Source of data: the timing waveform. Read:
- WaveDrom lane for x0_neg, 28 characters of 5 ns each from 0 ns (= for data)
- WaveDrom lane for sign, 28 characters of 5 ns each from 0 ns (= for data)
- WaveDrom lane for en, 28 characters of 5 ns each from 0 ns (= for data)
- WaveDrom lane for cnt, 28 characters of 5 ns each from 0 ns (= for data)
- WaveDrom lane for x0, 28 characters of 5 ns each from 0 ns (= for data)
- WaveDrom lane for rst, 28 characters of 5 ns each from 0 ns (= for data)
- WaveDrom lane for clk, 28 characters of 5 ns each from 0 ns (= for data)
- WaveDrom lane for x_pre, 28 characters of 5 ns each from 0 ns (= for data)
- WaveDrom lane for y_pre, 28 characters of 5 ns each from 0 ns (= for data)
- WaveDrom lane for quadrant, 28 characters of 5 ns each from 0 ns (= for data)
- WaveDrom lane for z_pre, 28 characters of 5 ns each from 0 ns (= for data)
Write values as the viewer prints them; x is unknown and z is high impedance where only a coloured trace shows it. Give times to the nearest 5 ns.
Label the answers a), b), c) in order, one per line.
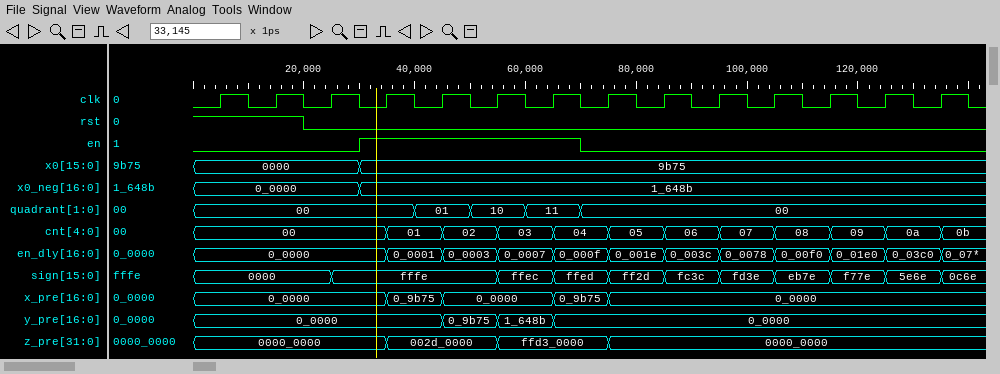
a) {name: 'x0_neg', wave: '=.....=.....................', data: '0_0000 1_648b'}
b) {name: 'sign', wave: '=....=.....=.=.=.=.=.=.=.=.=', data: '0000 fffe ffec ffed ff2d fc3c fd3e eb7e f77e 5e6e 0c6e'}
c) {name: 'en', wave: '0.....1.......0.............'}
d) {name: 'cnt', wave: '=......=.=.=.=.=.=.=.=.=.=.=', data: '00 01 02 03 04 05 06 07 08 09 0a 0b'}
e) {name: 'x0', wave: '=.....=.....................', data: '0000 9b75'}
f) {name: 'rst', wave: '1...0.......................'}
g) {name: 'clk', wave: '0101010101010101010101010101'}
h) {name: 'x_pre', wave: '=......=.=...=.=............', data: '0_0000 0_9b75 0_0000 0_9b75 0_0000'}
i) {name: 'y_pre', wave: '=........=.=.=..............', data: '0_0000 0_9b75 1_648b 0_0000'}
j) {name: 'quadrant', wave: '=.......=.=.=.=.............', data: '00 01 10 11 00'}
k) {name: 'z_pre', wave: '=......=...=...=............', data: '0000_0000 002d_0000 ffd3_0000 0000_0000'}
